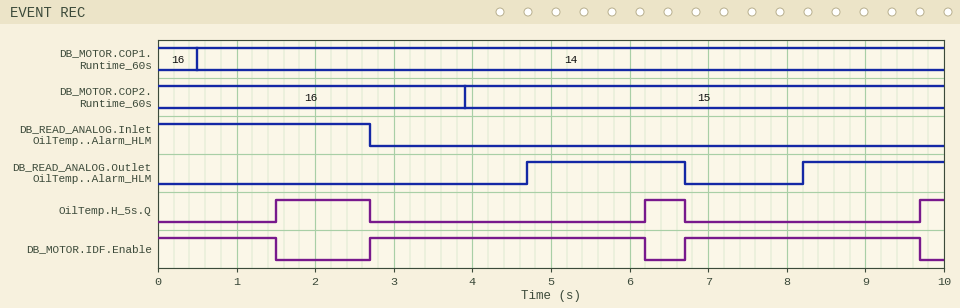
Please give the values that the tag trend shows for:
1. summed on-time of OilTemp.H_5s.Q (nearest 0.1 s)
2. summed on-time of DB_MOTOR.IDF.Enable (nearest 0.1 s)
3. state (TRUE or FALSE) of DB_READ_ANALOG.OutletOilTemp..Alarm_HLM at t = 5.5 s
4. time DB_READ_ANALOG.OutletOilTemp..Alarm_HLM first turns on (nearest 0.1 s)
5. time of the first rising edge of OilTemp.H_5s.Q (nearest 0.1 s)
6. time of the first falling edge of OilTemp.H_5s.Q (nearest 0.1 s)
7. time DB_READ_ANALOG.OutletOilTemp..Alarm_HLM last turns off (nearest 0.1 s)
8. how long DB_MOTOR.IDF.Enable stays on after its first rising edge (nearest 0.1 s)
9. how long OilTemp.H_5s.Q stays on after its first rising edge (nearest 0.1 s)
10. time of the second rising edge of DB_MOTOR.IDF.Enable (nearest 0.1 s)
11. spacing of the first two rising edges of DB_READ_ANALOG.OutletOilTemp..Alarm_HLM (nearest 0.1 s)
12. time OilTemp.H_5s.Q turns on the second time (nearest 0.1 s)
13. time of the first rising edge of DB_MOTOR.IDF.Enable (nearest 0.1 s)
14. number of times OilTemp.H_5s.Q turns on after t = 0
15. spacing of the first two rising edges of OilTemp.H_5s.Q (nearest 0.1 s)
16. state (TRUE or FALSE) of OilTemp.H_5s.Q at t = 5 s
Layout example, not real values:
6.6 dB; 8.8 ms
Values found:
2.0 s; 8.0 s; TRUE; 4.7 s; 1.5 s; 2.7 s; 6.7 s; 3.5 s; 1.2 s; 6.7 s; 3.5 s; 6.2 s; 2.7 s; 3; 4.7 s; FALSE
